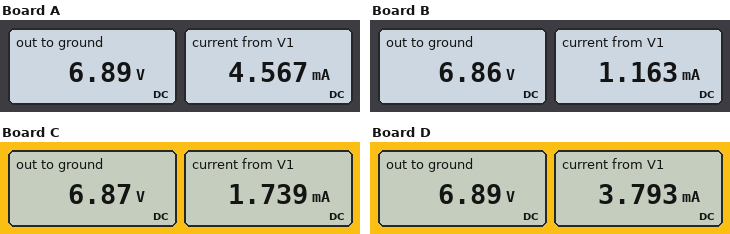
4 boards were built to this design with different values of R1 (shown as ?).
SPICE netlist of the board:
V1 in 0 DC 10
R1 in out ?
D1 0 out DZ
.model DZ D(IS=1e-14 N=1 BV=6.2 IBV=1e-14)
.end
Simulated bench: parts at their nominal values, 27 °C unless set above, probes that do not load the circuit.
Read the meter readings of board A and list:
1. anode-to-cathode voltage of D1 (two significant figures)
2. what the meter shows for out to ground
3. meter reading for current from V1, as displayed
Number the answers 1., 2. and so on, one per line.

1. -6.9 V
2. 6.89 V
3. 4.567 mA
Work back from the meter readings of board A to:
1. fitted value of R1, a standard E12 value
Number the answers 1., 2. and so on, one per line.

1. 680 Ω
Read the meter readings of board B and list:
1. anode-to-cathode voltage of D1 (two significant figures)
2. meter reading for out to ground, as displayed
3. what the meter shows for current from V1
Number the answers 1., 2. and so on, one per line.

1. -6.9 V
2. 6.86 V
3. 1.163 mA
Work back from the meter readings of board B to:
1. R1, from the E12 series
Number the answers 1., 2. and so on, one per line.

1. 2.7 kΩ
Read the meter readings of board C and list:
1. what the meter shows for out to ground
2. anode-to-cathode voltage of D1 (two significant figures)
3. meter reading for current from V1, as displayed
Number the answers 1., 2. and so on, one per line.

1. 6.87 V
2. -6.9 V
3. 1.739 mA
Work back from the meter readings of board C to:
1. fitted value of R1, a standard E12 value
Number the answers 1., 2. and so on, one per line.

1. 1.8 kΩ
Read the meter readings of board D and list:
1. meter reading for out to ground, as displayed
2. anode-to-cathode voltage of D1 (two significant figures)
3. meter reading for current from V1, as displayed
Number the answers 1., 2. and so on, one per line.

1. 6.89 V
2. -6.9 V
3. 3.793 mA
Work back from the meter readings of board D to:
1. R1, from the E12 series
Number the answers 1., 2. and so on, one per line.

1. 820 Ω
